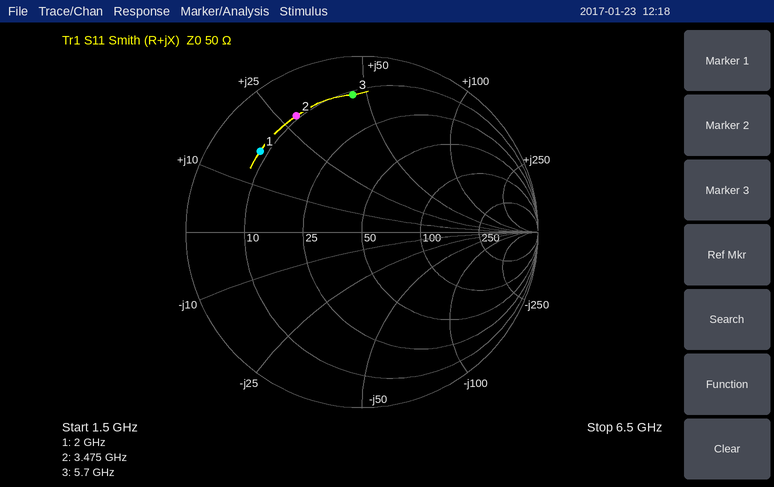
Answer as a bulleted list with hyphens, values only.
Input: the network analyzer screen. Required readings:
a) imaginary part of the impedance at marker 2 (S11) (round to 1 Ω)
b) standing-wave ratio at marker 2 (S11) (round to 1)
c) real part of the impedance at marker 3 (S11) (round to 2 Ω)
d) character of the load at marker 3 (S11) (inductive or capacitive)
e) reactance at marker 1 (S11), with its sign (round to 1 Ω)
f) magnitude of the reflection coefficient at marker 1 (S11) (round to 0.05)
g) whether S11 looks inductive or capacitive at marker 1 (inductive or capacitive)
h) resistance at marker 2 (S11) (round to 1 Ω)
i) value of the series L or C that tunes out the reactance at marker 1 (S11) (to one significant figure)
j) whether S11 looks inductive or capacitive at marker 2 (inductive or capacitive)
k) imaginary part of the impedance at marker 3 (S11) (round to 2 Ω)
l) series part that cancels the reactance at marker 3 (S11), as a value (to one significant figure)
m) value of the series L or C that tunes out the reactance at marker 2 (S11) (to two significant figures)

- +28 Ω
- 7
- 12 Ω
- inductive
- +17 Ω
- 0.75
- inductive
- 9 Ω
- 5 pF
- inductive
- +46 Ω
- 600 fF
- 1.6 pF
